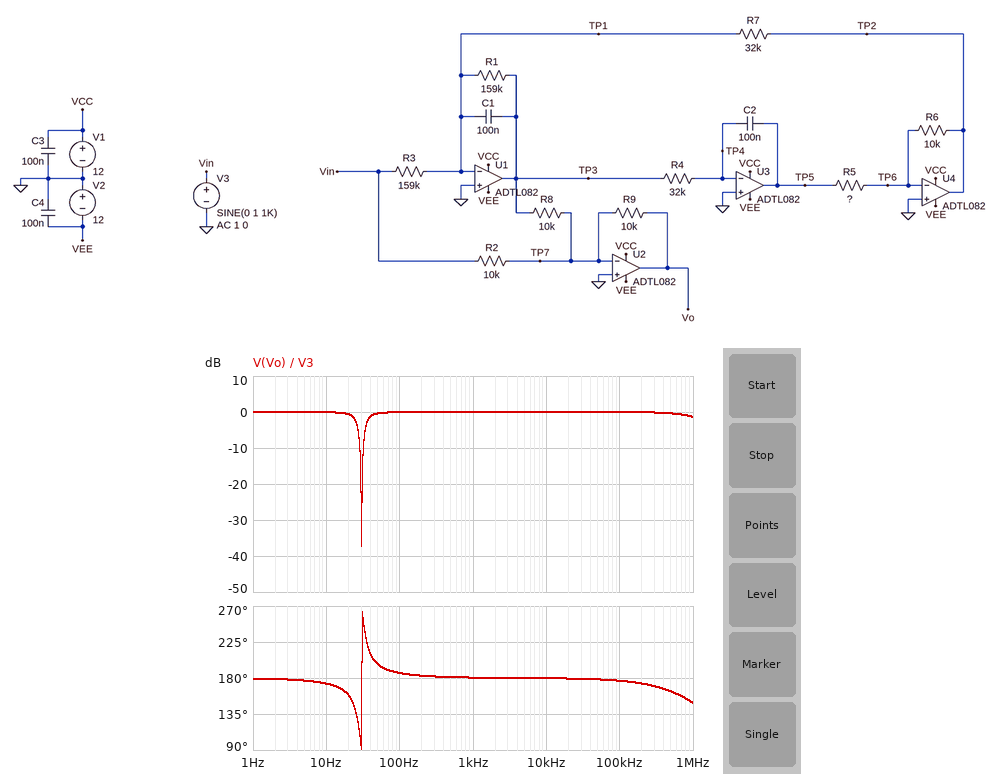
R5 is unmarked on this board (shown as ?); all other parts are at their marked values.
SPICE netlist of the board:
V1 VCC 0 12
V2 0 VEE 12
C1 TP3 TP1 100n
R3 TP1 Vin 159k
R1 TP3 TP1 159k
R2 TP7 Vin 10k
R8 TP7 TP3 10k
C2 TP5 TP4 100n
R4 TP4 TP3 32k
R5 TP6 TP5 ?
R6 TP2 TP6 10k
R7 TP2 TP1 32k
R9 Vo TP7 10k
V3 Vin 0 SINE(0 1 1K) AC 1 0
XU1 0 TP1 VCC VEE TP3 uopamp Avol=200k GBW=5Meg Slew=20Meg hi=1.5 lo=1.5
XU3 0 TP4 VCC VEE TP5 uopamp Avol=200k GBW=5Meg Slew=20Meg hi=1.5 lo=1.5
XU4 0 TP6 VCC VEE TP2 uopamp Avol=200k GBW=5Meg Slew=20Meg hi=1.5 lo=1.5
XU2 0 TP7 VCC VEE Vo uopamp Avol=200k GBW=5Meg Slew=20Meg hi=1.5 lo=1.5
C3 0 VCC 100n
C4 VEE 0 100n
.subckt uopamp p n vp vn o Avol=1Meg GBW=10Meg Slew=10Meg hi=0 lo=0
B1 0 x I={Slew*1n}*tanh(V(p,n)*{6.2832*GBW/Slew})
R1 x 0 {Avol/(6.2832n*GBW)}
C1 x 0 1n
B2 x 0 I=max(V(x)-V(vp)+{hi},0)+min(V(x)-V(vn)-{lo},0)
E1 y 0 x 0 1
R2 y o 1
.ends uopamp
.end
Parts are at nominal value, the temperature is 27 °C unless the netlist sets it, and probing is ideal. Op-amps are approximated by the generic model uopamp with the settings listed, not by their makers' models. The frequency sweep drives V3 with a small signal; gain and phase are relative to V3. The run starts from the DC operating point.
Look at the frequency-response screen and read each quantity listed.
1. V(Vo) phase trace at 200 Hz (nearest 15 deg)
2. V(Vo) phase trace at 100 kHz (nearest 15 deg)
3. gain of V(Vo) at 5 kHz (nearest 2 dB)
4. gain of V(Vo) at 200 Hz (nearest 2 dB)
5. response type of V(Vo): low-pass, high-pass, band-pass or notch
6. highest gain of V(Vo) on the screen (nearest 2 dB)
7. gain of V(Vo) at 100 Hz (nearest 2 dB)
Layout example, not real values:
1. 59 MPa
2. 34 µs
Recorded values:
1. 180 deg
2. 180 deg
3. 0 dB
4. 0 dB
5. notch
6. 0 dB
7. 0 dB
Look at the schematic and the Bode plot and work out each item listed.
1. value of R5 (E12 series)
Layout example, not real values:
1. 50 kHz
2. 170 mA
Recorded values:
1. 27 kΩ
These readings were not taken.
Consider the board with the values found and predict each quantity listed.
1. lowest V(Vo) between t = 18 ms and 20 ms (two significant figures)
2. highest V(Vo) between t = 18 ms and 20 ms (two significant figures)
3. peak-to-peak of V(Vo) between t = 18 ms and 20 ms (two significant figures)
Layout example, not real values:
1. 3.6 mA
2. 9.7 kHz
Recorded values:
1. -1.0 V
2. 1.0 V
3. 2.0 V
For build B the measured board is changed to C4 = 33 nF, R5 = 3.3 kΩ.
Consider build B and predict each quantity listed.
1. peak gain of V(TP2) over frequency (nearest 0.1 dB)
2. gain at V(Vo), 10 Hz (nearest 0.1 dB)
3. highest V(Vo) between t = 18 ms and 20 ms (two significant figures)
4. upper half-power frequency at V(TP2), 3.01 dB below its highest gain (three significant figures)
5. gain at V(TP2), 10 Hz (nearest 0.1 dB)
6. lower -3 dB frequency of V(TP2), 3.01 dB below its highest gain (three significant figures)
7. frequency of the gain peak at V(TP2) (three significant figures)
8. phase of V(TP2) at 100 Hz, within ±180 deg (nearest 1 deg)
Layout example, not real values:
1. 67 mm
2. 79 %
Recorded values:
1. 4.8 dB
2. 0 dB
3. 1.0 V
4. 91.2 Hz
5. -13.8 dB
6. 81.1 Hz
7. 86.3 Hz
8. 22 deg
